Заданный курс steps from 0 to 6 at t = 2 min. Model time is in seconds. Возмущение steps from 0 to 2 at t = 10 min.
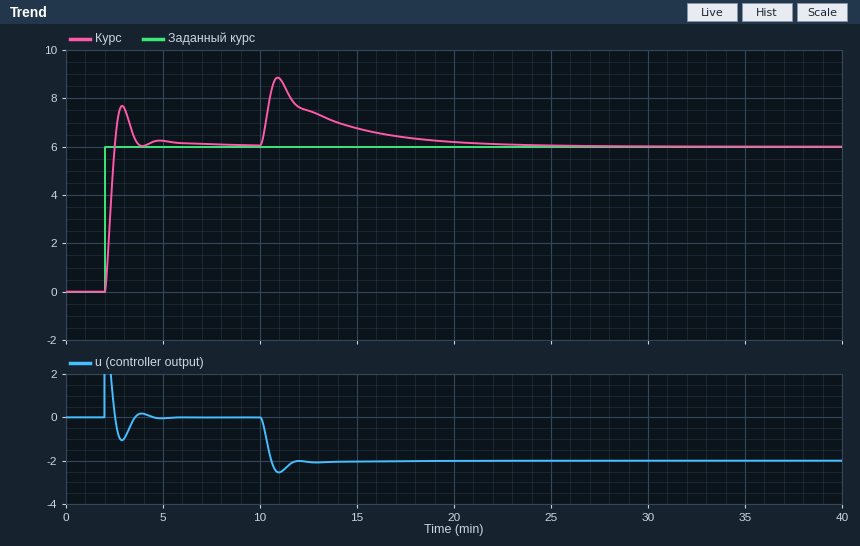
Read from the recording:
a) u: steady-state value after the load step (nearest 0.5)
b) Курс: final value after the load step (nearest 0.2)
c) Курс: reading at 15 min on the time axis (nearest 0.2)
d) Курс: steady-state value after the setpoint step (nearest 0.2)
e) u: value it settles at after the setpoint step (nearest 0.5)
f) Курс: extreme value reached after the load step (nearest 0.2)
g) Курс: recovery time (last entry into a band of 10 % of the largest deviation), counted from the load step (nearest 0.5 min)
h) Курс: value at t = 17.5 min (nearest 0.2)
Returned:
-2.0
6.0
6.8
6.0
0.0
8.8
8.5 min
6.4
